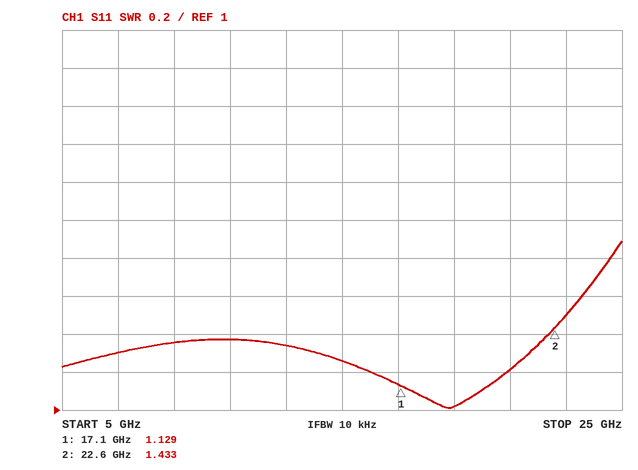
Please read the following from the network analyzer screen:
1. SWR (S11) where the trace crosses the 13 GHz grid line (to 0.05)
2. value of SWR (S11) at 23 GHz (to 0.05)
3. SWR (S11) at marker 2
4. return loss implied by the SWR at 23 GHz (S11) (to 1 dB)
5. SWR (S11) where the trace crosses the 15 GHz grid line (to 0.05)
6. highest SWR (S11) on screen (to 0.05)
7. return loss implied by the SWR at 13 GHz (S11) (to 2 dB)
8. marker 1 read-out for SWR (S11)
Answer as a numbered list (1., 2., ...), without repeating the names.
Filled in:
1. 1.35
2. 1.50
3. 1.433
4. 14 dB
5. 1.25
6. 1.90
7. 16 dB
8. 1.129
